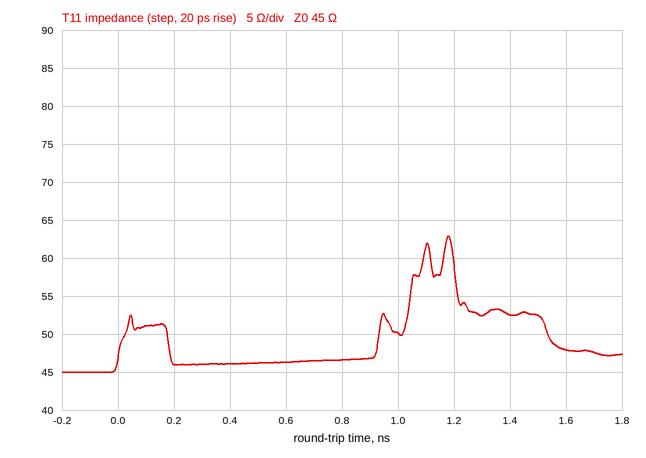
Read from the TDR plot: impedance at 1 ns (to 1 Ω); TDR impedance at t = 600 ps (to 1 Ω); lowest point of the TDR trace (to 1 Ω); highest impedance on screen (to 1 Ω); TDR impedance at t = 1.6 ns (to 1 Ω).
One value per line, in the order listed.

50 Ω
46 Ω
45 Ω
63 Ω
48 Ω
